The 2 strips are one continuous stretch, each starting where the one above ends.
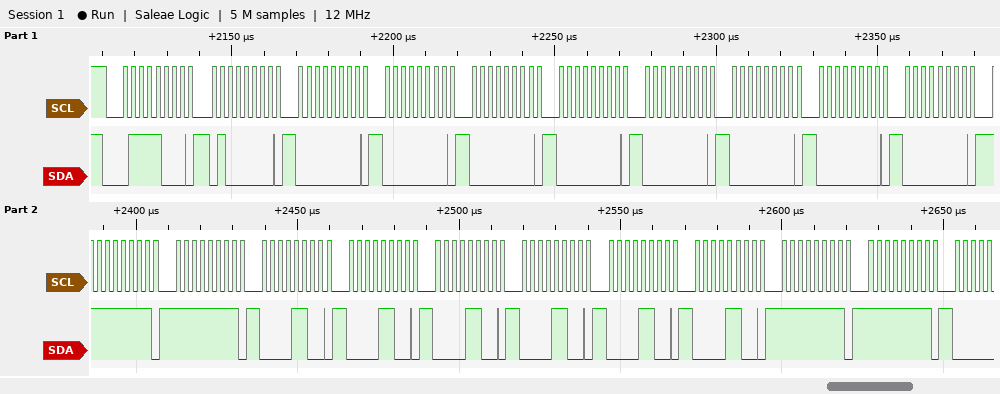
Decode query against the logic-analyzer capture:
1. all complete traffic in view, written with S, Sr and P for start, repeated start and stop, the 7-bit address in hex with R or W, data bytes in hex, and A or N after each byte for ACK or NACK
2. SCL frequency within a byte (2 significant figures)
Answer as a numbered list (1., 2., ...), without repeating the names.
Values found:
1. S 3CW A 40 A 00 A 00 A 00 A 00 A 00 A 00 A 00 A 00 A FF A FF A 0C A 0C A 0C A 0C A 0C A 0C A FF A FF A
2. 400 kHz
